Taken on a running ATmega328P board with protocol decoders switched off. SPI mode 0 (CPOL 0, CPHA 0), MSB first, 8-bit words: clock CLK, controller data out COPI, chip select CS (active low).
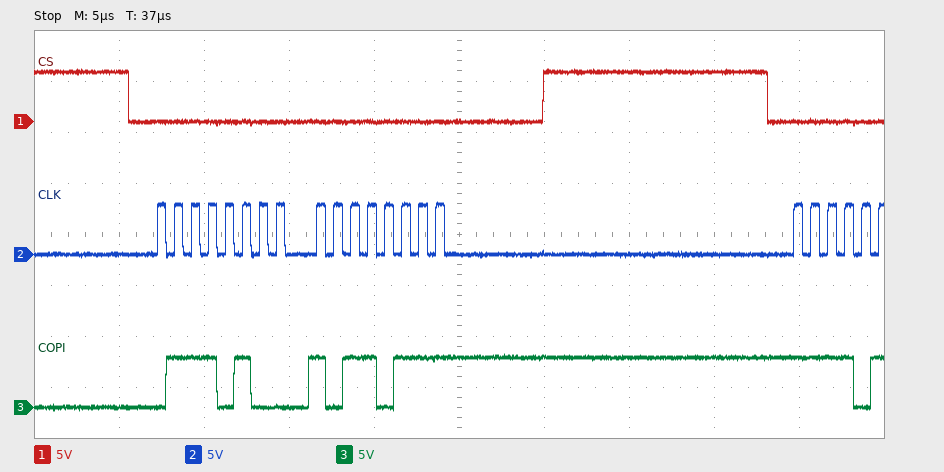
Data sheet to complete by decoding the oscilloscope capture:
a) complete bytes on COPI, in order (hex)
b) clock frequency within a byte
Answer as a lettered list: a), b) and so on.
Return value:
a) 0x74 0xB7
b) 1 MHz
